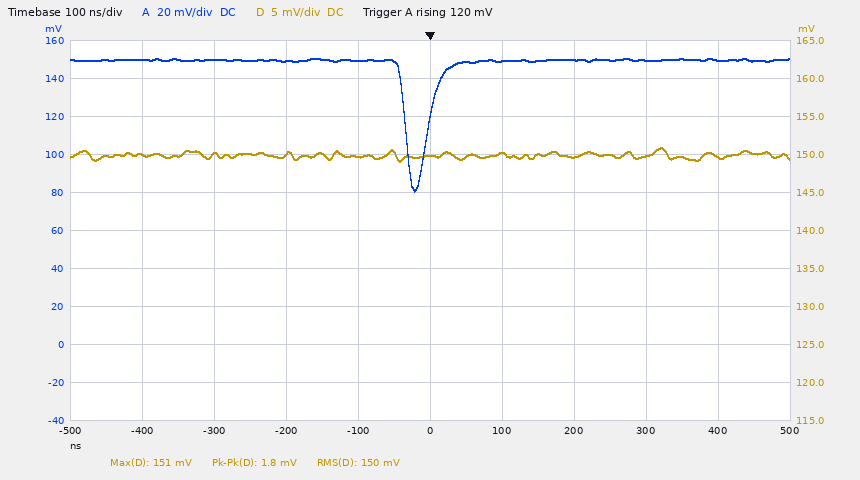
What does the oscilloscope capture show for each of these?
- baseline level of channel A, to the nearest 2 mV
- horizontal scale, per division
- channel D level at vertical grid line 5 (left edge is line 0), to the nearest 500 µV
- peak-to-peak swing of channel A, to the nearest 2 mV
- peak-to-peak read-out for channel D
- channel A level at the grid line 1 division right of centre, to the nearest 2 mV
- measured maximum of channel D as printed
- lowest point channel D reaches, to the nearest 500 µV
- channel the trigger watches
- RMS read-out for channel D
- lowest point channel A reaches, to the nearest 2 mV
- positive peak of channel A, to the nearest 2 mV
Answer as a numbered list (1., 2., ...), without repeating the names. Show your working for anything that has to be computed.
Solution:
1. 150 mV
2. 100 ns
3. 150.0 mV
4. 150 mV − (80 mV) = 70 mV
5. 1.8 mV
6. 150 mV
7. 151 mV
8. 149.0 mV
9. channel A
10. 150 mV
11. 80 mV
12. 150 mV
